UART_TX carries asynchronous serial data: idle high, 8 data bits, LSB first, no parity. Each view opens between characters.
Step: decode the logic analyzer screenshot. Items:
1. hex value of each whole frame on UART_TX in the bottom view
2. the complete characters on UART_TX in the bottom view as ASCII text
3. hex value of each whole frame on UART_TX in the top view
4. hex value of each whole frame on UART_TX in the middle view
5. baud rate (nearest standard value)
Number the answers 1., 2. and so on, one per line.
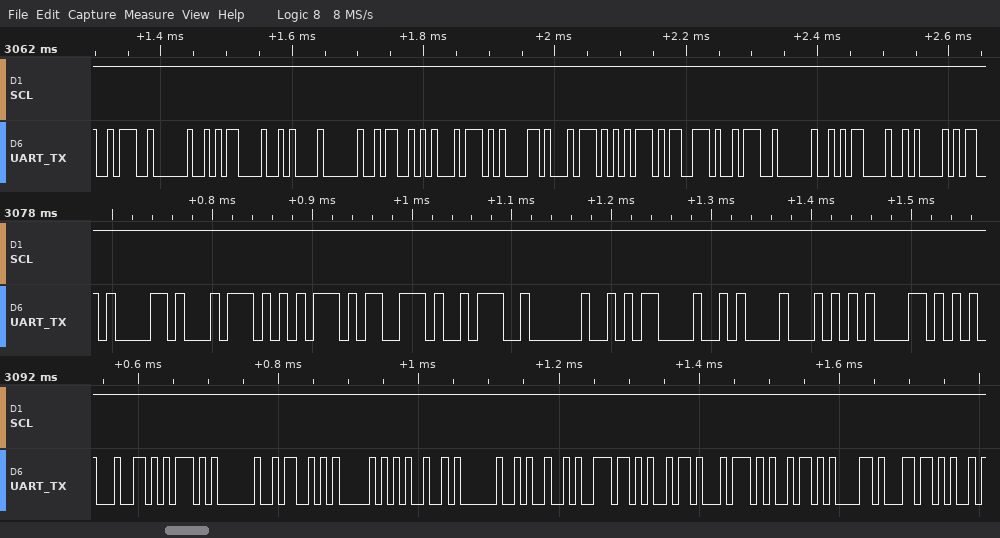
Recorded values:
1. 64, 5D, 20, 53, 50, 49, 20, 49, 6E, 69, 74, 69, 61, 6C
2. "d] SPI Initial"
3. 3A, 20, 0D, 0A, 20, 53, 74, 61, 74, 75, 73, 3A, 20, 0D, 0A
4. 61, 74, 75, 73, 3A, 20, 0D, 0A, 54, 58
5. 115200 baud
